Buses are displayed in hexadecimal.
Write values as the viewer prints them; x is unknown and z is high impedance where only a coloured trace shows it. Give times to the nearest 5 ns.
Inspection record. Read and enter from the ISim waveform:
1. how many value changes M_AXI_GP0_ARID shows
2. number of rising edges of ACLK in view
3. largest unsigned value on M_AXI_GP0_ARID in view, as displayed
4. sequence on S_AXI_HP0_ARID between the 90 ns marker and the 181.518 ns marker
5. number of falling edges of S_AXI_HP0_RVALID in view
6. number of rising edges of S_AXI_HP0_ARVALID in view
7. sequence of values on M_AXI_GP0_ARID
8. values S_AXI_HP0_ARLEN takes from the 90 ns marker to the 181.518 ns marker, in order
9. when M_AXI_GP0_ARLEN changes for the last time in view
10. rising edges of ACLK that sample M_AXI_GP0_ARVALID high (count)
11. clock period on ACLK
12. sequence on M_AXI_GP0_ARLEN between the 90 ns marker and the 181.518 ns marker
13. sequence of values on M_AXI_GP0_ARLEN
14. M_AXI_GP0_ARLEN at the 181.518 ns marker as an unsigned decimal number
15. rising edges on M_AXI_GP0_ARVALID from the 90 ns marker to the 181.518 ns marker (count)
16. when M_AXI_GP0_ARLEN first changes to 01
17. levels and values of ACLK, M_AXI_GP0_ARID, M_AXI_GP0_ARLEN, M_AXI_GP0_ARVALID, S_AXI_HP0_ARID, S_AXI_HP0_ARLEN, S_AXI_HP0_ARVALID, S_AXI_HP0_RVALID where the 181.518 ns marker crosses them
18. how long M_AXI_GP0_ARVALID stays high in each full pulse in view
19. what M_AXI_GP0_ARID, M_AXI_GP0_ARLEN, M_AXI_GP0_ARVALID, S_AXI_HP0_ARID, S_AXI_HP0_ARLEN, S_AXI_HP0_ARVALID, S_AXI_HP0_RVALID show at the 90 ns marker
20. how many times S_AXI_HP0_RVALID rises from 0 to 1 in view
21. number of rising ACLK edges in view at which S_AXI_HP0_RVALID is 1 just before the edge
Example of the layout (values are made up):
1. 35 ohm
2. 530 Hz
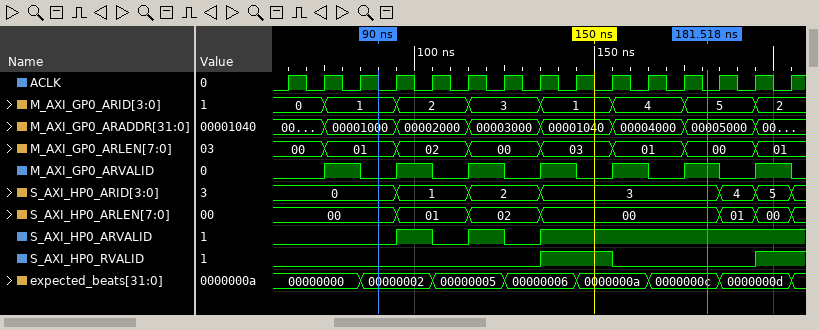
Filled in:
1. 7
2. 15
3. 5
4. 0, 1, 2, 3
5. 1
6. 3
7. 0, 1, 2, 3, 1, 4, 5, 2
8. 00, 01, 02, 00
9. 195 ns
10. 7
11. 10 ns
12. 01, 02, 00, 03, 01, 00
13. 00, 01, 02, 00, 03, 01, 00, 01
14. 0
15. 5
16. 75 ns
17. ACLK=0, M_AXI_GP0_ARID=5, M_AXI_GP0_ARLEN=00, M_AXI_GP0_ARVALID=1, S_AXI_HP0_ARID=3, S_AXI_HP0_ARLEN=00, S_AXI_HP0_ARVALID=1, S_AXI_HP0_RVALID=0
18. 10 ns, 10 ns, 10 ns, 10 ns, 10 ns, 10 ns, 10 ns
19. M_AXI_GP0_ARID=1, M_AXI_GP0_ARLEN=01, M_AXI_GP0_ARVALID=0, S_AXI_HP0_ARID=0, S_AXI_HP0_ARLEN=00, S_AXI_HP0_ARVALID=0, S_AXI_HP0_RVALID=0
20. 2
21. 3
